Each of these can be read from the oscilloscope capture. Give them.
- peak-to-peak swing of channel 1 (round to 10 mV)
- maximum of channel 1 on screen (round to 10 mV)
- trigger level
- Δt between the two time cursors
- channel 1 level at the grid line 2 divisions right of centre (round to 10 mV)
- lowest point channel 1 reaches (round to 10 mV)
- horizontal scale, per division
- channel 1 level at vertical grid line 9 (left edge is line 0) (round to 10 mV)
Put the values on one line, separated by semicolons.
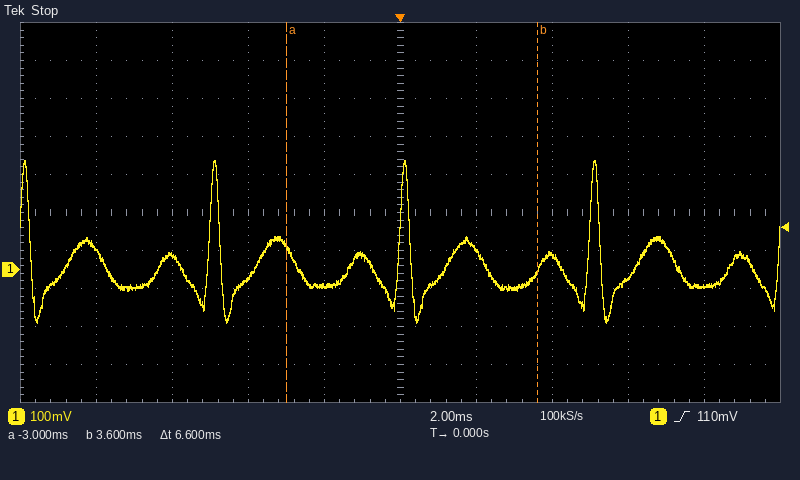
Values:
430 mV; 290 mV; 110 mV; 6.6 ms; 40 mV; -140 mV; 2 ms; -40 mV
